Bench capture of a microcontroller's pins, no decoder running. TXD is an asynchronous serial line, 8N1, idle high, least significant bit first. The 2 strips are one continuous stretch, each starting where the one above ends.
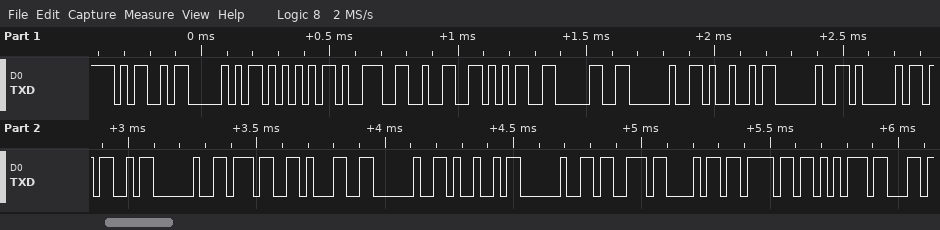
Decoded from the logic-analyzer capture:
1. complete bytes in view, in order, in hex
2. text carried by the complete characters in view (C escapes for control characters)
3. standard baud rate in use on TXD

4D 50 55 39 32 35 30 20 49 20 41 4D 20 37 31 20 49 20 73 68 6F 75
"MPU9250 I AM 71 I shou"
38400 baud
